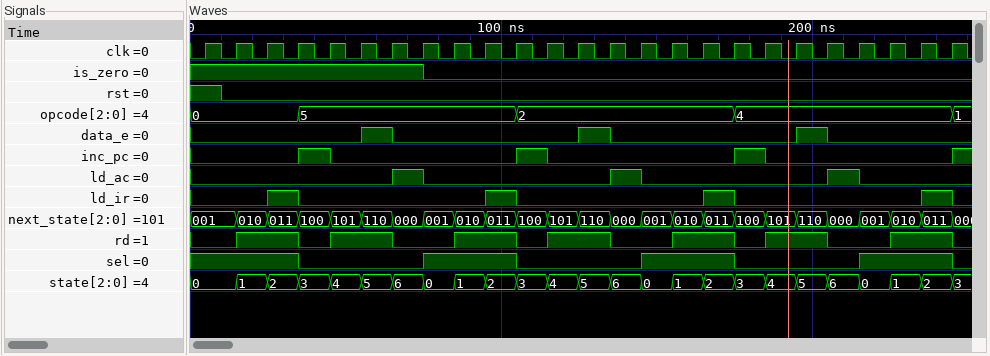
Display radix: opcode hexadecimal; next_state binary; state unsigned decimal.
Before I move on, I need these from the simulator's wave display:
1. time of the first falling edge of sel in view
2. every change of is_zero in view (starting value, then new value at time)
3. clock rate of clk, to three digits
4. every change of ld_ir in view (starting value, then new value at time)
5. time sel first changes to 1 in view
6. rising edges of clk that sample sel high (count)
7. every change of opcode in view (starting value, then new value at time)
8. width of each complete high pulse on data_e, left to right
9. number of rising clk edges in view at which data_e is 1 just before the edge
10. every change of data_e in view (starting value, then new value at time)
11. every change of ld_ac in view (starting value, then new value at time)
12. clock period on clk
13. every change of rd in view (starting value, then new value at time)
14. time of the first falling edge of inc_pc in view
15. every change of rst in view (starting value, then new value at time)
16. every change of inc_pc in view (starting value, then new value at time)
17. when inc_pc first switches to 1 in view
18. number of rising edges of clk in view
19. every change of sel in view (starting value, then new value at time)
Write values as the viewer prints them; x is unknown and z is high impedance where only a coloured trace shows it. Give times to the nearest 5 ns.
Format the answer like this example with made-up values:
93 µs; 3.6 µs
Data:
35 ns; 1, 0 at 75 ns; 100 MHz; 0, 1 at 25 ns, 0 at 35 ns, 1 at 95 ns, 0 at 105 ns, 1 at 165 ns, 0 at 175 ns, 1 at 235 ns, 0 at 245 ns; 75 ns; 13; 0, 5 at 35 ns, 2 at 105 ns, 4 at 175 ns, 1 at 245 ns; 10 ns, 10 ns, 10 ns; 3; 0, 1 at 55 ns, 0 at 65 ns, 1 at 125 ns, 0 at 135 ns, 1 at 195 ns, 0 at 205 ns; 0, 1 at 65 ns, 0 at 75 ns, 1 at 135 ns, 0 at 145 ns, 1 at 205 ns, 0 at 215 ns; 10 ns; 0, 1 at 15 ns, 0 at 35 ns, 1 at 45 ns, 0 at 65 ns, 1 at 85 ns, 0 at 105 ns, 1 at 115 ns, 0 at 135 ns, 1 at 155 ns, 0 at 175 ns, 1 at 185 ns, 0 at 205 ns, 1 at 225 ns, 0 at 245 ns; 45 ns; 1, 0 at 10 ns; 0, 1 at 35 ns, 0 at 45 ns, 1 at 105 ns, 0 at 115 ns, 1 at 175 ns, 0 at 185 ns, 1 at 245 ns; 35 ns; 25; 1, 0 at 35 ns, 1 at 75 ns, 0 at 105 ns, 1 at 145 ns, 0 at 175 ns, 1 at 215 ns, 0 at 245 ns
